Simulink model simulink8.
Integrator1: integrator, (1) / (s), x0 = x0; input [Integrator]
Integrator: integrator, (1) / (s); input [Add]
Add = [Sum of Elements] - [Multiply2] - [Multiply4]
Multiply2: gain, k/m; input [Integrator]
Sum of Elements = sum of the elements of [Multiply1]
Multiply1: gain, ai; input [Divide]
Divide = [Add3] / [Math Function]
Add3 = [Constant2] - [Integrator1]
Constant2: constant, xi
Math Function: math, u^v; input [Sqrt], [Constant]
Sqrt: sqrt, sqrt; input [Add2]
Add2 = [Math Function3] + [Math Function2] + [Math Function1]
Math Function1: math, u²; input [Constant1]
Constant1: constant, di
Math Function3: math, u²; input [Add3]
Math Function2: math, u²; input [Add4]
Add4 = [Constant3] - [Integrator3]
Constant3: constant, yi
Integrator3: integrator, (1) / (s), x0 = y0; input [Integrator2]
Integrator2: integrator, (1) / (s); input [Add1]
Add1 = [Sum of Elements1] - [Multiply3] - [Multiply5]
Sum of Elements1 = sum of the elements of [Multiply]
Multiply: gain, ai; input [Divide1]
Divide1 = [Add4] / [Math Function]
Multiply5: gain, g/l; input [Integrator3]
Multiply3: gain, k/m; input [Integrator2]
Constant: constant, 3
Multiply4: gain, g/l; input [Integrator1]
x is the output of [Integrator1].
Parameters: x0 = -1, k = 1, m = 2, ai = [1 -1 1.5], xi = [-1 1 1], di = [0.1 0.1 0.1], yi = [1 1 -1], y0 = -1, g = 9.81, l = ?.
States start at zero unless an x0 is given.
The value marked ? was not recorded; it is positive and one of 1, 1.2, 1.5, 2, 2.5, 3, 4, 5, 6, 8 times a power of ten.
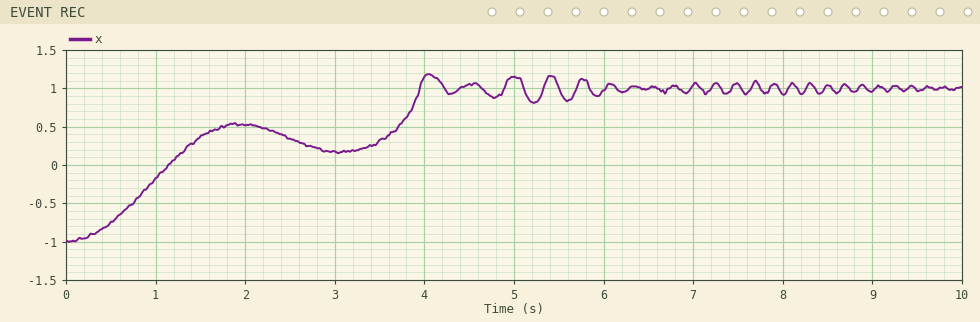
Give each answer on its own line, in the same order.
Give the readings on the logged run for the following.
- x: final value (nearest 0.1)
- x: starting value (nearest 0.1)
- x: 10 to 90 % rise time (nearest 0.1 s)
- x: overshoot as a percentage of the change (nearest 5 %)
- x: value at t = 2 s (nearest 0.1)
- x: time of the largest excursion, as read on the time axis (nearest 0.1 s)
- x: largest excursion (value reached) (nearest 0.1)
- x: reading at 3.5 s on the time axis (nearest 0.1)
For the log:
1.0
-1.0
3.4 s
10 %
0.5
4.1 s
1.2
0.3
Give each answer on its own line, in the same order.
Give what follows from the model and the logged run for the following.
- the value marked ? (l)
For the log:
5
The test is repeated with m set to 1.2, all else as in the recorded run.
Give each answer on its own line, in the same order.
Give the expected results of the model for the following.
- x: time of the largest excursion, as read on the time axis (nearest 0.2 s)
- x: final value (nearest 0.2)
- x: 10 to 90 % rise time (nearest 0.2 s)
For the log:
4.2 s
1.0
3.6 s
